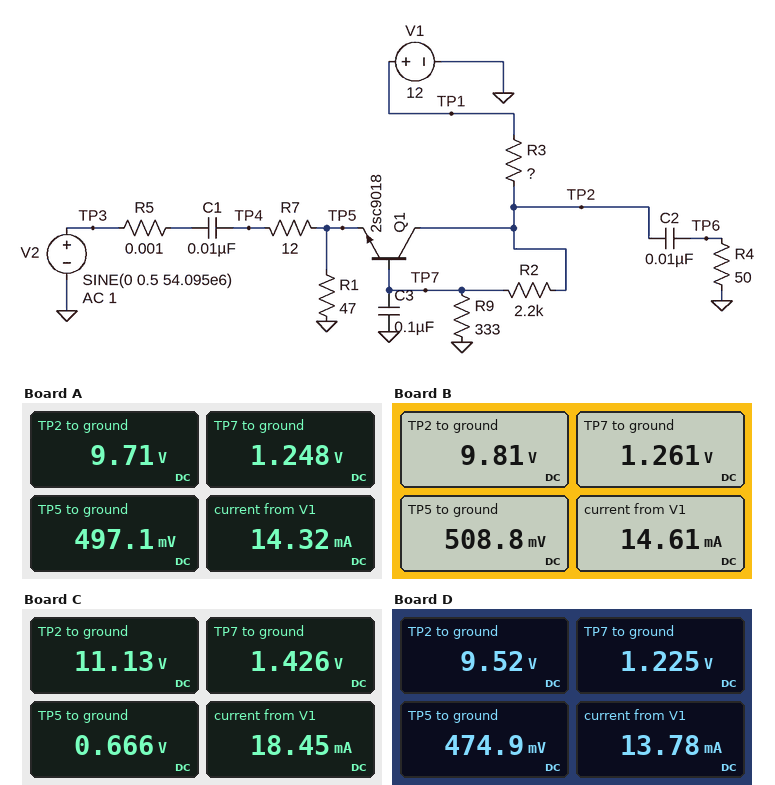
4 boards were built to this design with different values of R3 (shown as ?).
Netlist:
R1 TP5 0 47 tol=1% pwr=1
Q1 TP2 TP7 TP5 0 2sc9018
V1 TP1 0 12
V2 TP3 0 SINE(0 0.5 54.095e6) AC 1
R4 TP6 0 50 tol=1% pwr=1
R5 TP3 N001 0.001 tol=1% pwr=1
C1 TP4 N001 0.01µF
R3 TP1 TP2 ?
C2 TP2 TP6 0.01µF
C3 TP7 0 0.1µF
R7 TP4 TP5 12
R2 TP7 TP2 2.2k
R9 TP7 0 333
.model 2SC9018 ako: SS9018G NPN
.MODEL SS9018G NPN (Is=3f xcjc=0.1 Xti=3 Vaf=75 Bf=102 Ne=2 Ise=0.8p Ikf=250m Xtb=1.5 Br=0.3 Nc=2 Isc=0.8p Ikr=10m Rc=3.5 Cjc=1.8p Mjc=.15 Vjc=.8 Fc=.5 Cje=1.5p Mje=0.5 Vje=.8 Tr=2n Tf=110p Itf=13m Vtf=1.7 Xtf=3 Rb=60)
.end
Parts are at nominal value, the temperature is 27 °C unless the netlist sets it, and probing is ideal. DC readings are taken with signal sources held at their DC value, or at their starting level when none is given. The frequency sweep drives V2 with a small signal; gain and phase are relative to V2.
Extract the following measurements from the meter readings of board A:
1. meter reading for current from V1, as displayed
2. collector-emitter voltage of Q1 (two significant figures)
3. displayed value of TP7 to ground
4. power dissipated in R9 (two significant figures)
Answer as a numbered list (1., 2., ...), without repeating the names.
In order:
1. 14.32 mA
2. 9.2 V
3. 1.248 V
4. 4.7 mW
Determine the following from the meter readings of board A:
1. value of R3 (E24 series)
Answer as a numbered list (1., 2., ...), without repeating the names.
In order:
1. 160 Ω
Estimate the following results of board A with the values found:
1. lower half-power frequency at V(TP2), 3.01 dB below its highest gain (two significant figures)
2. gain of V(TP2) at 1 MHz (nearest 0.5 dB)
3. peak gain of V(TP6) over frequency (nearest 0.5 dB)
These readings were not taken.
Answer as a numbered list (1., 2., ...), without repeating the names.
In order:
1. 970 kHz
2. 4.5 dB
3. 7.5 dB
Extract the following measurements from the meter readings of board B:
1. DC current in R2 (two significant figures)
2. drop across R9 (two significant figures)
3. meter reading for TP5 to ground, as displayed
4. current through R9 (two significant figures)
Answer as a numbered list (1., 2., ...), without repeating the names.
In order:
1. 3.9 mA
2. 1.3 V
3. 508.8 mV
4. 3.8 mA
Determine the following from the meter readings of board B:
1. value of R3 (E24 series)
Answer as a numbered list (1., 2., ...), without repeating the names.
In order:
1. 150 Ω
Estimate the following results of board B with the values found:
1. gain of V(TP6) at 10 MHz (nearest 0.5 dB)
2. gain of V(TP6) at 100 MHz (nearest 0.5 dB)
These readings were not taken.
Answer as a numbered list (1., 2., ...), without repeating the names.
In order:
1. 7.0 dB
2. 6.5 dB
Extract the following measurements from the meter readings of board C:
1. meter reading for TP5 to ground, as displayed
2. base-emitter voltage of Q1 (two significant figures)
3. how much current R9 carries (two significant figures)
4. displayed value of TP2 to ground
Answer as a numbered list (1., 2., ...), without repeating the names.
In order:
1. 0.666 V
2. 760 mV
3. 4.3 mA
4. 11.13 V
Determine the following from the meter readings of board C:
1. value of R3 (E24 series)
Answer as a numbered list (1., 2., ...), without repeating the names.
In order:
1. 47 Ω
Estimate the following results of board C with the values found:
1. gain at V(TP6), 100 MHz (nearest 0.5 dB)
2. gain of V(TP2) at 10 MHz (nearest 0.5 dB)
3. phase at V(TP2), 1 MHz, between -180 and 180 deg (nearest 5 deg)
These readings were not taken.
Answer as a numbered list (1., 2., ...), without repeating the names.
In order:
1. 3.0 dB
2. 4.0 dB
3. 40 deg
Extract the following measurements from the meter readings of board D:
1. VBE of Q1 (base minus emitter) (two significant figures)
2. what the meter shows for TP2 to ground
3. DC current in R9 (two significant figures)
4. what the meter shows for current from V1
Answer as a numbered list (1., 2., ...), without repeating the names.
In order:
1. 750 mV
2. 9.52 V
3. 3.7 mA
4. 13.78 mA
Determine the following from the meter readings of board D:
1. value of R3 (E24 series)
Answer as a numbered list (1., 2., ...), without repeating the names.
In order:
1. 180 Ω
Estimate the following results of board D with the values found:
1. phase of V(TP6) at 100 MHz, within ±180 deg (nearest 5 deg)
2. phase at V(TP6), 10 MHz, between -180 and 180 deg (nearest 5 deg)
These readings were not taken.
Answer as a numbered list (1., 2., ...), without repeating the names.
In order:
1. -25 deg
2. 5 deg
